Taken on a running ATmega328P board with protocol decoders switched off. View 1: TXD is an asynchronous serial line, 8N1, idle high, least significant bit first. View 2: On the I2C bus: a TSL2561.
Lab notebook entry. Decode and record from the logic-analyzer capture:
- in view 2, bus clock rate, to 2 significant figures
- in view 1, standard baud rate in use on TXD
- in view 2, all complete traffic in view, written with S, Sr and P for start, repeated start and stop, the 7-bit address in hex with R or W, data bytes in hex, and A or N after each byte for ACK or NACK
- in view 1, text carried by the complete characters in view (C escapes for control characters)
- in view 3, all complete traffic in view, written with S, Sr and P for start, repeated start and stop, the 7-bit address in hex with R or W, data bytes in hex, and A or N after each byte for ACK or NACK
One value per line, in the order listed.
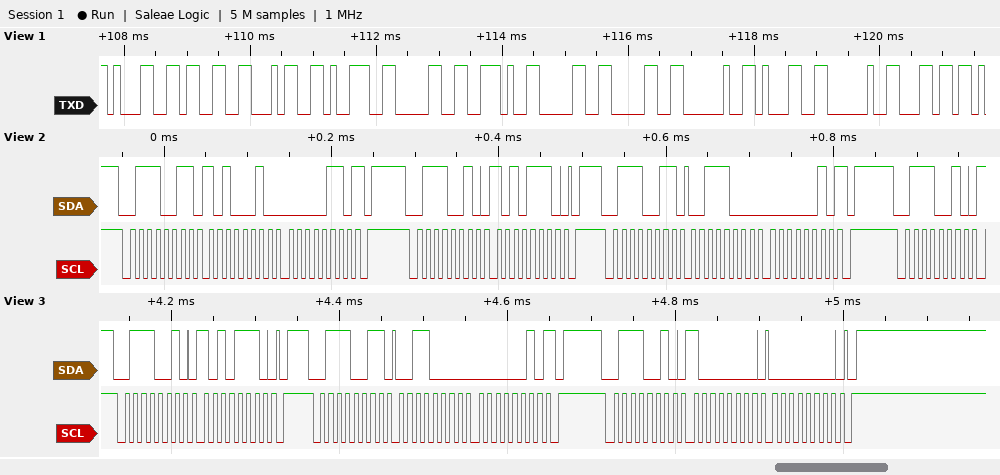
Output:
100 kHz
9600 baud
S 39R A A2 A 06 N P S 39W A AE A P S 39R A 38 A 02 N P S 39W A
"13490.00 1 l"
S 39W A AE A P S 39R A 30 A 02 N P S 39W A 80 A 00 A P
